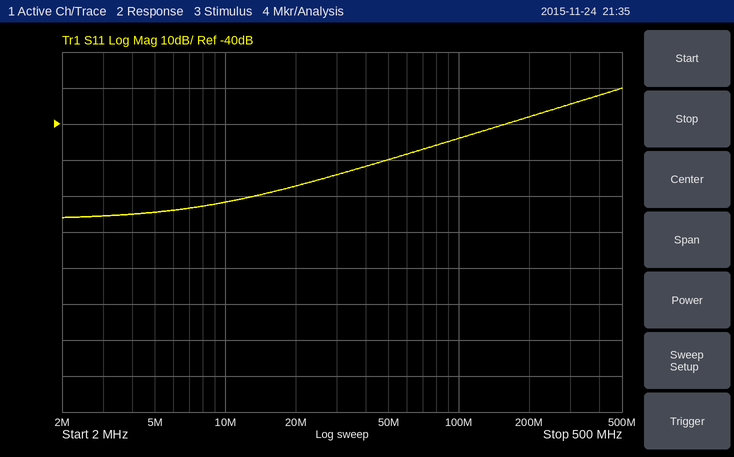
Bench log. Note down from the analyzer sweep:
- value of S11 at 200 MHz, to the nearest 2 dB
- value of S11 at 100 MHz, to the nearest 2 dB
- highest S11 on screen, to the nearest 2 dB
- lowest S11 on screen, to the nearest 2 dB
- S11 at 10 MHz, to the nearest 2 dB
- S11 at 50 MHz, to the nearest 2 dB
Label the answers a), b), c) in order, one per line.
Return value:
a) -38 dB
b) -44 dB
c) -30 dB
d) -66 dB
e) -62 dB
f) -50 dB
